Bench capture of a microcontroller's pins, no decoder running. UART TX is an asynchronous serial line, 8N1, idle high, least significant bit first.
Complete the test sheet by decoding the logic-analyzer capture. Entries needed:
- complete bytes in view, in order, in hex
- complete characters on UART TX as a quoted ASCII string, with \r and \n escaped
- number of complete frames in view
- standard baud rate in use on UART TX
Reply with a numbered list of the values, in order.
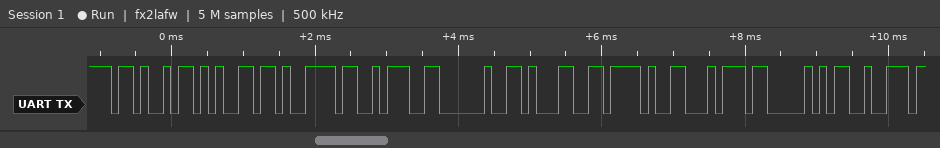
1. 4B 65 79 3A 20 31 2F 74 50 72
2. "Key: 1/tPr"
3. 10
4. 9600 baud
